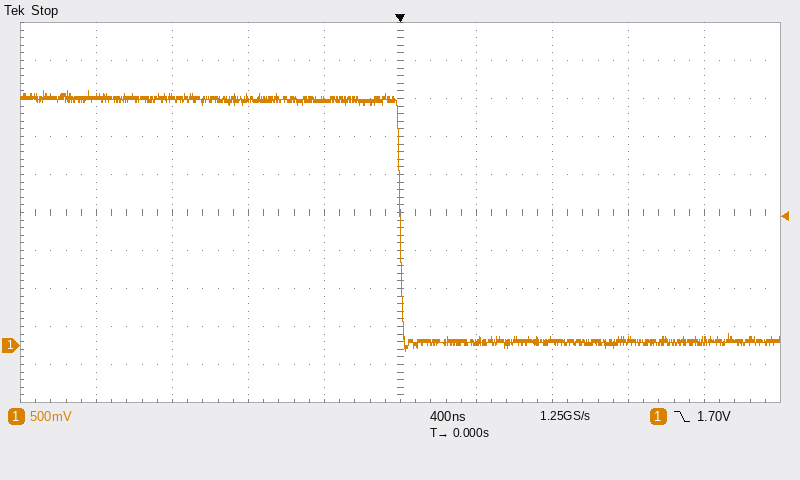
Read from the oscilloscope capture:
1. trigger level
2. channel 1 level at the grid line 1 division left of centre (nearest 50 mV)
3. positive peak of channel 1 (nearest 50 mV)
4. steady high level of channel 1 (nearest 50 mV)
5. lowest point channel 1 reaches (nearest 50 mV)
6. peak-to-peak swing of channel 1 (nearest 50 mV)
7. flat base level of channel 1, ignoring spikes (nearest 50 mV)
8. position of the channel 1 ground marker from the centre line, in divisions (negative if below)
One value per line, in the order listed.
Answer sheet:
1.70 V
3.25 V
3.35 V
3.25 V
-100 mV
3.45 V
50 mV
-3.5 div
